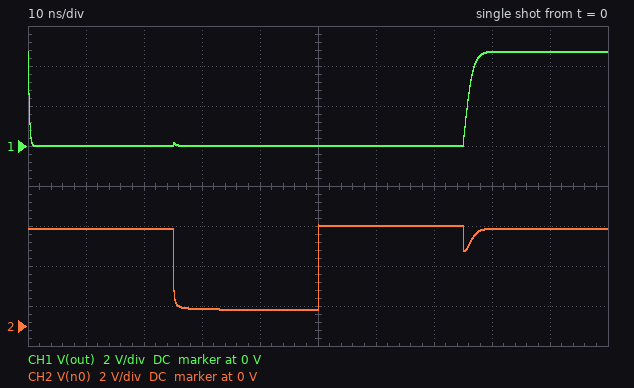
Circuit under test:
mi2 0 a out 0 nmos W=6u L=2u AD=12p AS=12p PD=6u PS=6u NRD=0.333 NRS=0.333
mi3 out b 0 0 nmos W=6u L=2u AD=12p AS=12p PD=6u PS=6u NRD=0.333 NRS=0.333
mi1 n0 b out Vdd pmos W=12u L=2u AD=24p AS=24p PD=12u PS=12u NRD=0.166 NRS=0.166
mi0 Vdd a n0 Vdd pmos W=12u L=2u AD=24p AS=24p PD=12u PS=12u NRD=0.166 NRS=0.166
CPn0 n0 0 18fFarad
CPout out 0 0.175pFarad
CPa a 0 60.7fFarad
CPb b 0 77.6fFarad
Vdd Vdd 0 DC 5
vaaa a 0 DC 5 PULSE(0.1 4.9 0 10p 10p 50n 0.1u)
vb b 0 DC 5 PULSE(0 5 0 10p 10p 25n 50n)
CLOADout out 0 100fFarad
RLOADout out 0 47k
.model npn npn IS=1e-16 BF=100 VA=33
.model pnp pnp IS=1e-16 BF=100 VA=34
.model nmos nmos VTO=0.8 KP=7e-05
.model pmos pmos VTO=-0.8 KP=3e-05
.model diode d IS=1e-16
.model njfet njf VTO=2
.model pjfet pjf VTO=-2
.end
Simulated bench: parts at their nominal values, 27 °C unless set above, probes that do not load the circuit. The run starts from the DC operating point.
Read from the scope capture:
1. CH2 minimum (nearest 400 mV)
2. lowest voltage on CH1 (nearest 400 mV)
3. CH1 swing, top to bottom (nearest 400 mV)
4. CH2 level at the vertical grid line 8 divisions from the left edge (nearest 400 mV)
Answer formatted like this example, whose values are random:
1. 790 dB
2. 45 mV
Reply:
1. 800 mV
2. 0 V
3. 4.8 V
4. 4.8 V
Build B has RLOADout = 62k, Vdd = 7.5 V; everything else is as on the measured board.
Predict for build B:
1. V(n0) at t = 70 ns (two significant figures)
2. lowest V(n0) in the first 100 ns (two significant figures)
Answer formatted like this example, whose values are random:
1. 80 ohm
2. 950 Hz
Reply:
1. 7.3 V
2. 2.6 V
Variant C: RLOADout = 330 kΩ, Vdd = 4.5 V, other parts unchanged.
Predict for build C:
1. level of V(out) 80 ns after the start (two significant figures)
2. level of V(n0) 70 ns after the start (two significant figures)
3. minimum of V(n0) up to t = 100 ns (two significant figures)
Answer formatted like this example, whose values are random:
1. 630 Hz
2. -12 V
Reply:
1. 4.4 V
2. 4.5 V
3. 810 mV
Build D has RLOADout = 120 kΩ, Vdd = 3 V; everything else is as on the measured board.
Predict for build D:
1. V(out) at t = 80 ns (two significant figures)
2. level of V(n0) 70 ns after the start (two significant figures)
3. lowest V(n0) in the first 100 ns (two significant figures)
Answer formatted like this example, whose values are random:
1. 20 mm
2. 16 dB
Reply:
1. 2.6 V
2. 3.0 V
3. 810 mV
